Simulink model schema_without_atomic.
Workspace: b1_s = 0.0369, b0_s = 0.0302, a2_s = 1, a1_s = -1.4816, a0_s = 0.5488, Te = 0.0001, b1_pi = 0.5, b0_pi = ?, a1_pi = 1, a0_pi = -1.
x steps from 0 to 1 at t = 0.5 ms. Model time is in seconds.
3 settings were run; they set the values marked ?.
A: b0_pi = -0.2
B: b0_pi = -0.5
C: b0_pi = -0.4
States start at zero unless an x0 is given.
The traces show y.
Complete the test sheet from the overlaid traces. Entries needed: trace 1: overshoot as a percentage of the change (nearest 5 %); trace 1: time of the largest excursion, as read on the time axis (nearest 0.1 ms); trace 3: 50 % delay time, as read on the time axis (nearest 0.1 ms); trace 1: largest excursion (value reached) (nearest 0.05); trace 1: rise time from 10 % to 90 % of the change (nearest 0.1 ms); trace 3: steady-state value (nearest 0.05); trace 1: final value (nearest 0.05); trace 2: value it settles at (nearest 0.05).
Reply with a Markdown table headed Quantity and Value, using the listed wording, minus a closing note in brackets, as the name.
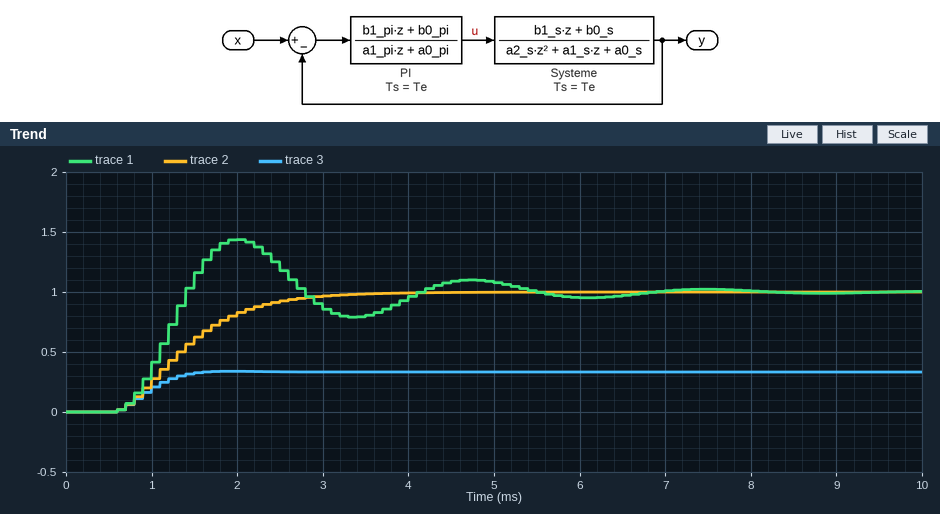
| Quantity | Value |
|---|---|
| trace 1: overshoot as a percentage of the change | 45 % |
| trace 1: time of the largest excursion, as read on the time axis | 2.0 ms |
| trace 3: 50 % delay time, as read on the time axis | 1.0 ms |
| trace 1: largest excursion (value reached) | 1.45 |
| trace 1: rise time from 10 % to 90 % of the change | 0.6 ms |
| trace 3: steady-state value | 0.35 |
| trace 1: final value | 1.00 |
| trace 2: value it settles at | 1.00 |
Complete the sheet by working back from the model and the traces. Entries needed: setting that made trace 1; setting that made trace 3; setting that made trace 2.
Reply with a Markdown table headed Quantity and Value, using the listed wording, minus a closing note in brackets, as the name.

| Quantity | Value |
|---|---|
| setting that made trace 1 | A |
| setting that made trace 3 | B |
| setting that made trace 2 | C |
